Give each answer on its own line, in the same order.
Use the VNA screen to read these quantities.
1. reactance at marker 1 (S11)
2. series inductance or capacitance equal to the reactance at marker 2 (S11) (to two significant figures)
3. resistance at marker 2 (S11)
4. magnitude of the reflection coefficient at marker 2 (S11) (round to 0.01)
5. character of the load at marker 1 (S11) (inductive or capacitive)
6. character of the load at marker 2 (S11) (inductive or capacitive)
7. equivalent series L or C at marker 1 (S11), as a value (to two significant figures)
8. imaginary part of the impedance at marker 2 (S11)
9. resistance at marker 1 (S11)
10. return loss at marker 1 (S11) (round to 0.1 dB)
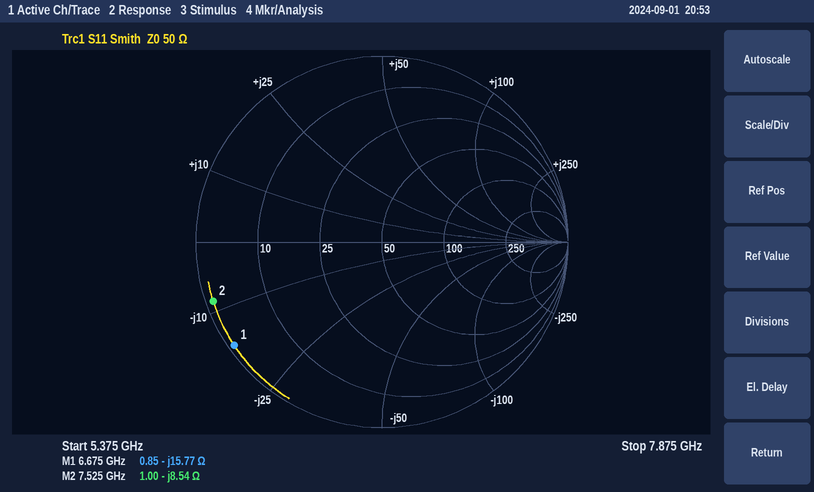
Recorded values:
-15.77 Ω
2.5 pF
1.00 Ω
0.96
capacitive
capacitive
1.5 pF
-8.54 Ω
0.85 Ω
0.3 dB
